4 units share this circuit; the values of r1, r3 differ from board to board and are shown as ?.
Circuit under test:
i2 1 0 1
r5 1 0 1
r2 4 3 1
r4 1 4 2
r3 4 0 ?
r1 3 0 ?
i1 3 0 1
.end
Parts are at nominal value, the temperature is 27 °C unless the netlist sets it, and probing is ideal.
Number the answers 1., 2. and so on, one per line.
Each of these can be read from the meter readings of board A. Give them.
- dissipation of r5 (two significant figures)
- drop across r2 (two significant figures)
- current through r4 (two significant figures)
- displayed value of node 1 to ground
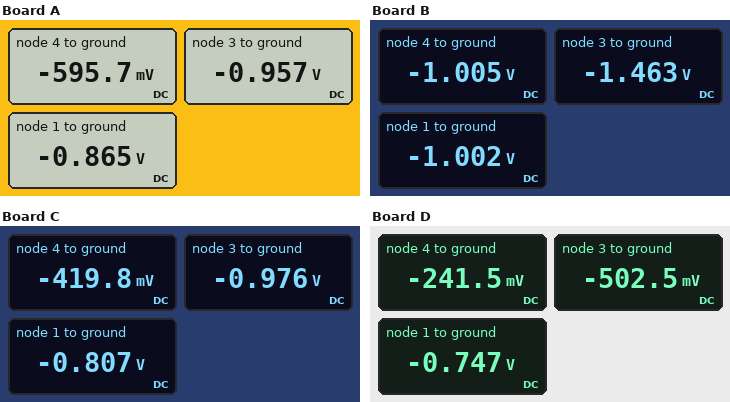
1. 750 mW
2. 360 mV
3. 130 mA
4. -0.865 V
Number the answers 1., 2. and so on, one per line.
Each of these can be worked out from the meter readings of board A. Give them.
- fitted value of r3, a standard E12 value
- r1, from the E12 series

1. 1.2 Ω
2. 1.5 Ω
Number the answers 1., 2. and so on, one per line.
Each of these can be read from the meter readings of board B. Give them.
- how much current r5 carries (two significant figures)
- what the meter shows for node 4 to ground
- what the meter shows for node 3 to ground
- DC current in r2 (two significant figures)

1. 1.0 A
2. -1.005 V
3. -1.463 V
4. 460 mA
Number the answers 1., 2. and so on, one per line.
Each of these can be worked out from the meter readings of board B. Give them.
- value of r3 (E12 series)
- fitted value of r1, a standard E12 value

1. 2.2 Ω
2. 2.7 Ω
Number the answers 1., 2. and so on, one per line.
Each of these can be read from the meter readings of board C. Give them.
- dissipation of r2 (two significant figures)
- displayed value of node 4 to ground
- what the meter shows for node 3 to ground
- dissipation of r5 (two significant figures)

1. 310 mW
2. -419.8 mV
3. -0.976 V
4. 650 mW
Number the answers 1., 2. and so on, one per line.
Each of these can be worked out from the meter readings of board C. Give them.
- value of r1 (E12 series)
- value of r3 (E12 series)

1. 2.2 Ω
2. 0.56 Ω
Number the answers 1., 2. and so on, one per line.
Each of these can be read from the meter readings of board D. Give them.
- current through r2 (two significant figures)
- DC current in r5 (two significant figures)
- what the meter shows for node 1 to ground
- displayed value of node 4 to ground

1. 260 mA
2. 750 mA
3. -0.747 V
4. -241.5 mV
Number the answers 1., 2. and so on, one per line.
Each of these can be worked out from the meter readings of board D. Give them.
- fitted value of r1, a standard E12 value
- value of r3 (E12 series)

1. 0.68 Ω
2. 0.47 Ω
